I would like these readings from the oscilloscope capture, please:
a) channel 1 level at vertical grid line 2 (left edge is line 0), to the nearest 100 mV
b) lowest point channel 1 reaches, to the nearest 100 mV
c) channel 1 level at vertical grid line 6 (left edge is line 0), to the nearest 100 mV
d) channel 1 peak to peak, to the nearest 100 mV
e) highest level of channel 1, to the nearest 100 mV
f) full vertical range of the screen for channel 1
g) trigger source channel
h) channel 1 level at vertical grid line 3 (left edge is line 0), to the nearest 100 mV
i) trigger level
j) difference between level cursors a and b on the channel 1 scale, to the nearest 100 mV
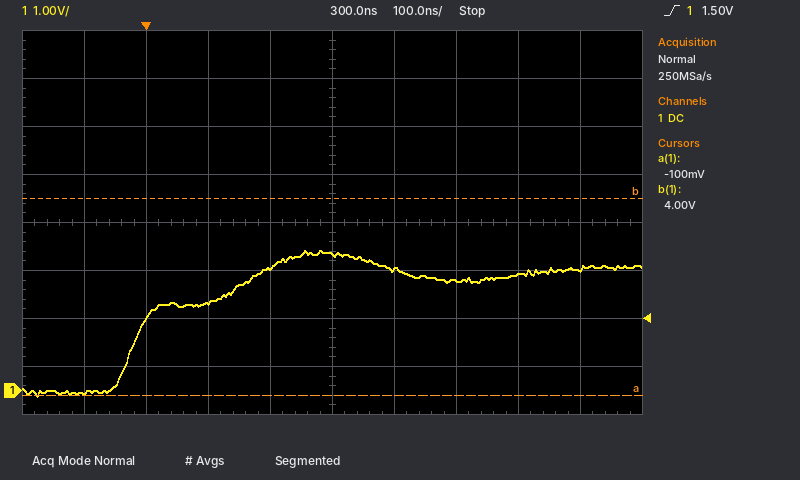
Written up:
1.5 V
-100 mV
2.5 V
3.0 V
2.9 V
8 V
channel 1
1.8 V
1.50 V
4.1 V
